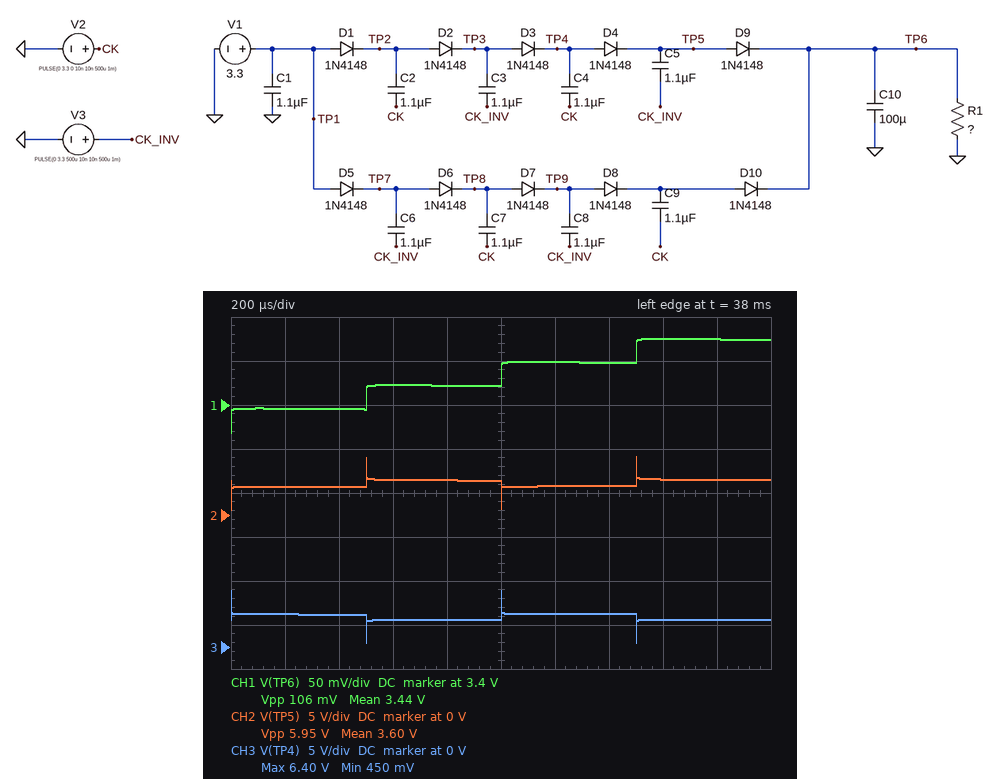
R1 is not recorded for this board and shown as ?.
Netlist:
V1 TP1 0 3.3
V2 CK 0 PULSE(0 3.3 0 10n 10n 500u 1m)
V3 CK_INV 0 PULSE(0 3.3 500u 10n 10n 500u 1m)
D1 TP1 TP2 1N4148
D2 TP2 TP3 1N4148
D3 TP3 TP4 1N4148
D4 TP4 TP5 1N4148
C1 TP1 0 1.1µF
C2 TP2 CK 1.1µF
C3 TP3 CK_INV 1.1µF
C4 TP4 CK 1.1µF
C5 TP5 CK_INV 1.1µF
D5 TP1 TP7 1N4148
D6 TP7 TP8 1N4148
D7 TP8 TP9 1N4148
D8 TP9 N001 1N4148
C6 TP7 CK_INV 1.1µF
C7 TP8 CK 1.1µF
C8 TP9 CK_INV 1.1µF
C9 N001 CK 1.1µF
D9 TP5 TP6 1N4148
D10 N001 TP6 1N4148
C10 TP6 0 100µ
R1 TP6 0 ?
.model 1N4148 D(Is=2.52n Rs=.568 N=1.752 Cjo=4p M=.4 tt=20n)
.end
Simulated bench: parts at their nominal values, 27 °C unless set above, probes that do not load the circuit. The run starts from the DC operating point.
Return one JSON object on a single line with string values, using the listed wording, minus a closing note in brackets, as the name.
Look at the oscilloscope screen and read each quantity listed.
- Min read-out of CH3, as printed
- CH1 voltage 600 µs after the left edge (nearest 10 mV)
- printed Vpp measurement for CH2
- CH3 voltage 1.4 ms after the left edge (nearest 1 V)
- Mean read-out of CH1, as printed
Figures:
{"Min read-out of CH3, as printed": "450 mV", "CH1 voltage 600 µs after the left edge": "3.42 V", "printed Vpp measurement for CH2": "5.95 V", "CH3 voltage 1.4 ms after the left edge": "4 V", "Mean read-out of CH1, as printed": "3.44 V"}
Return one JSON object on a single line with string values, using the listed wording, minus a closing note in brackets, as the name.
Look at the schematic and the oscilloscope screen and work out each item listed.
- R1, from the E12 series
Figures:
{"R1, from the E12 series": "6.8 kΩ"}
